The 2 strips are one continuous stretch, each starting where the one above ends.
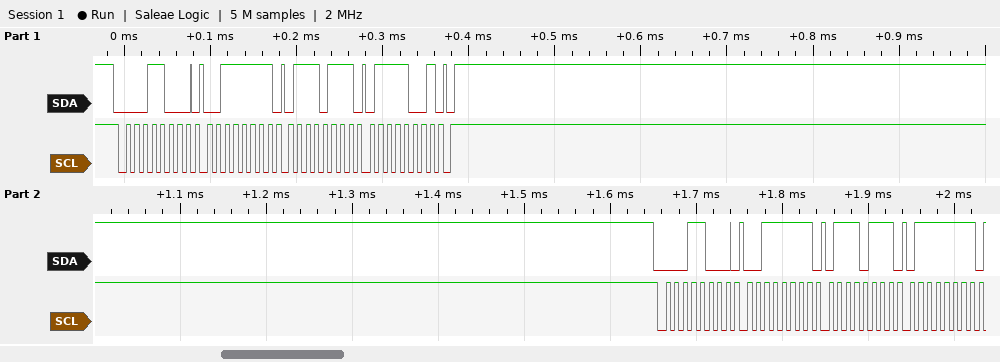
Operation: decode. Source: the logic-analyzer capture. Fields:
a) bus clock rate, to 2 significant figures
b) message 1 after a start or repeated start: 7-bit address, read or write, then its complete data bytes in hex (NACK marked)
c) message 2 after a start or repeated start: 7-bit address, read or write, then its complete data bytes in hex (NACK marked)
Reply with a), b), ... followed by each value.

a) 100 kHz
b) 0x0C write: 3F 77 79
c) 0x0C write: 3F 77 7F
